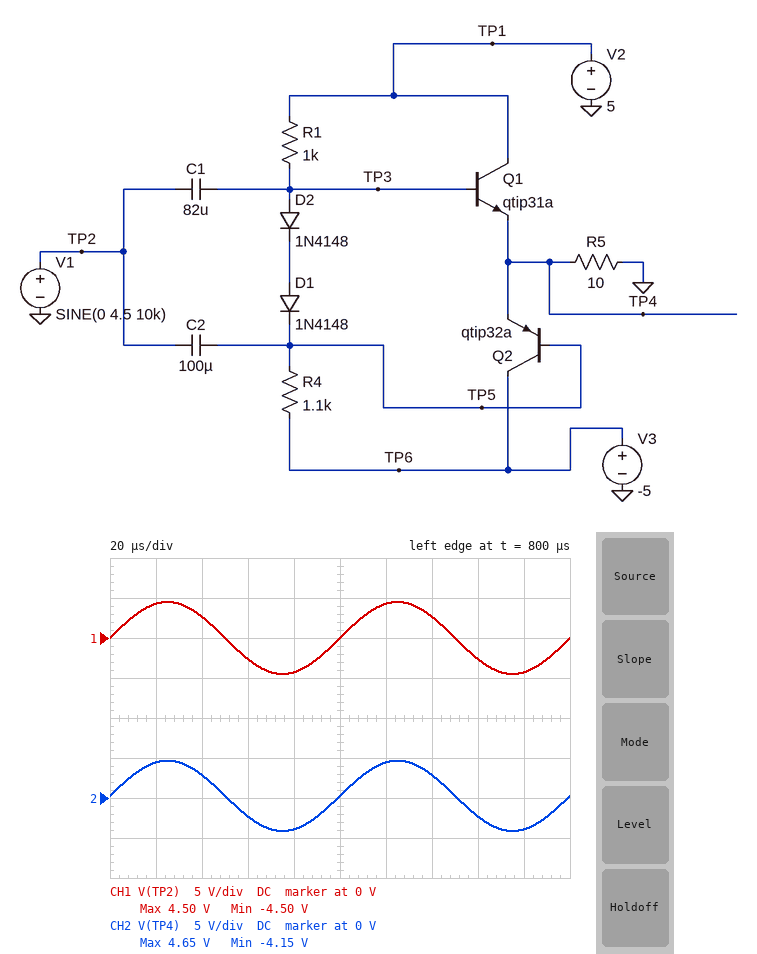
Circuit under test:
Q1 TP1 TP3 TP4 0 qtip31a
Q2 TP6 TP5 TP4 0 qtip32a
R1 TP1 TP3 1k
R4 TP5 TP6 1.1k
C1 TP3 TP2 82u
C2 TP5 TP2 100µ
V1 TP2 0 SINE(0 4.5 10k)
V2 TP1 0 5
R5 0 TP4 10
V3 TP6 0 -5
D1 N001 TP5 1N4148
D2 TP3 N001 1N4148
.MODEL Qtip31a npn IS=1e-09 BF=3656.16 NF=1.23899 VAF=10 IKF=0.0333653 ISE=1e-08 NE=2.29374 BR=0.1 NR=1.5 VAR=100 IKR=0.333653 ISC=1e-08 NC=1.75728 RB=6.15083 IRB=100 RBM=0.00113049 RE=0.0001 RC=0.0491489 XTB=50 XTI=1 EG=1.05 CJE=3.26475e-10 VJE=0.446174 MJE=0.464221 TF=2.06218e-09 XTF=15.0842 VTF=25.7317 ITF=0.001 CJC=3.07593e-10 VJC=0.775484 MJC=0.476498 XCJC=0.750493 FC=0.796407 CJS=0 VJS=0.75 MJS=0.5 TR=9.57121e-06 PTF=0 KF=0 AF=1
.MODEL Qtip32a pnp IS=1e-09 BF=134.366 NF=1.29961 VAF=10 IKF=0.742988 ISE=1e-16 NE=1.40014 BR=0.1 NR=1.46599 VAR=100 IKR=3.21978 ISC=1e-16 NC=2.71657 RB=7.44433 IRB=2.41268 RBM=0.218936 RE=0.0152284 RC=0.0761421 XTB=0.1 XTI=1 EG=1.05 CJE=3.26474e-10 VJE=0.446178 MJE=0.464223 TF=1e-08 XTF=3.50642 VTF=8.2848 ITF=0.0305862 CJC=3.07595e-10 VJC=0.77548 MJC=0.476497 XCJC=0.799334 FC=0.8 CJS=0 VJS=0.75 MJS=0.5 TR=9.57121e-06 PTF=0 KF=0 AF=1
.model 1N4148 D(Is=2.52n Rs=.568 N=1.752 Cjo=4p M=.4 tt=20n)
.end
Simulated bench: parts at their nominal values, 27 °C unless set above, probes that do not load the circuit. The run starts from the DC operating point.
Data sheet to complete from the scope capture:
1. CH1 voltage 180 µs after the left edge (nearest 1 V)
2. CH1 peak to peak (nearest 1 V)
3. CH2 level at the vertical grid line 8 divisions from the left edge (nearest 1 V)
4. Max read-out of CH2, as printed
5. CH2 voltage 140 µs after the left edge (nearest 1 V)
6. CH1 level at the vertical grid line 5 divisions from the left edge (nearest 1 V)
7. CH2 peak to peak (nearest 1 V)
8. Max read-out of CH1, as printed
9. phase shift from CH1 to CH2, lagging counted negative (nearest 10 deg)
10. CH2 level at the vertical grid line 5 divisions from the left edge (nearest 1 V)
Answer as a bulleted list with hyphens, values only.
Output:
- -4 V
- 9 V
- -2 V
- 4.65 V
- 3 V
- 0 V
- 9 V
- 4.50 V
- 0 deg
- 0 V
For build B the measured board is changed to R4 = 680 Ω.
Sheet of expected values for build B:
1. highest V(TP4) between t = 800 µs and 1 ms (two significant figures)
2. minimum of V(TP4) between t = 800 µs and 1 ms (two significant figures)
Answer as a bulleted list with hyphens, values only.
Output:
- 3.9 V
- -4.8 V
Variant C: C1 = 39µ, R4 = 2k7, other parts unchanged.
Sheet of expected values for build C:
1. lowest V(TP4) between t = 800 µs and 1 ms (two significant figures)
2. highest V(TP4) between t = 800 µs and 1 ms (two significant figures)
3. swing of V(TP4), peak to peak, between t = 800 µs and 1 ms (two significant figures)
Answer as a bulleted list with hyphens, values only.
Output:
- -2.9 V
- 4.9 V
- 7.8 V
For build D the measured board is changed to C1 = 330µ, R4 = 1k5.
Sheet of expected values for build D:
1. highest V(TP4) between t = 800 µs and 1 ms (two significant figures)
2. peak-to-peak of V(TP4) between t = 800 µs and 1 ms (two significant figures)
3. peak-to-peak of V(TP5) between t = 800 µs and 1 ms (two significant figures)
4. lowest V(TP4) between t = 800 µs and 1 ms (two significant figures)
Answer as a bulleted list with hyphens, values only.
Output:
- 4.8 V
- 8.5 V
- 9.0 V
- -3.7 V
